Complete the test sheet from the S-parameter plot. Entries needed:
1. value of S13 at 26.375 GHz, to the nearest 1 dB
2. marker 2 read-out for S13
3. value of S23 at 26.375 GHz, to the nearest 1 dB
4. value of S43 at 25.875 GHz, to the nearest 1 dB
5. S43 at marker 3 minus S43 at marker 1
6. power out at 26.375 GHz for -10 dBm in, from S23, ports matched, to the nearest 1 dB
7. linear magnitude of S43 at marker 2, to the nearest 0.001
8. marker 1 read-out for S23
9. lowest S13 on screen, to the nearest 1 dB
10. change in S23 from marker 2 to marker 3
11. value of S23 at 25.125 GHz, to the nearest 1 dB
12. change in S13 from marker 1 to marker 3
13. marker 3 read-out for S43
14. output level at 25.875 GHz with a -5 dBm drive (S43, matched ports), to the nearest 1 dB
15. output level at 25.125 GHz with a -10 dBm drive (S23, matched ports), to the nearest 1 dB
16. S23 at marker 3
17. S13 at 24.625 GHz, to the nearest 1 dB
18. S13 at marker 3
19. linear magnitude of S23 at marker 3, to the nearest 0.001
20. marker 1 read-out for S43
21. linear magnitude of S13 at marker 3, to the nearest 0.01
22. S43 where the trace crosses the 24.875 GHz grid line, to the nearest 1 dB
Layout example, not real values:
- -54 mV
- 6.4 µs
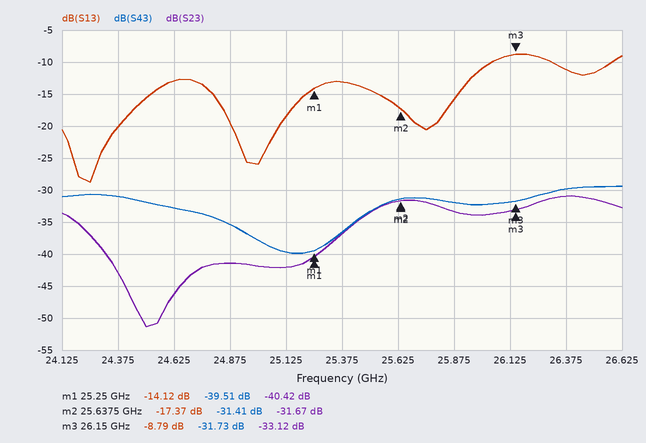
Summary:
- -11 dB
- -17.37 dB
- -31 dB
- -32 dB
- 7.78 dB
- -41 dBm
- 0.027
- -40.42 dB
- -29 dB
- -1.45 dB
- -42 dB
- 5.33 dB
- -31.73 dB
- -37 dBm
- -52 dBm
- -33.12 dB
- -13 dB
- -8.79 dB
- 0.022
- -39.51 dB
- 0.36
- -35 dB
